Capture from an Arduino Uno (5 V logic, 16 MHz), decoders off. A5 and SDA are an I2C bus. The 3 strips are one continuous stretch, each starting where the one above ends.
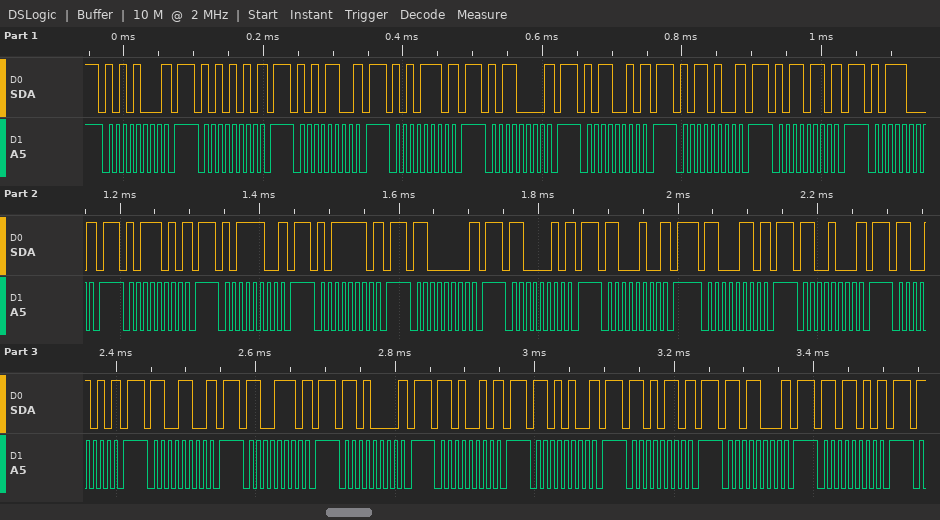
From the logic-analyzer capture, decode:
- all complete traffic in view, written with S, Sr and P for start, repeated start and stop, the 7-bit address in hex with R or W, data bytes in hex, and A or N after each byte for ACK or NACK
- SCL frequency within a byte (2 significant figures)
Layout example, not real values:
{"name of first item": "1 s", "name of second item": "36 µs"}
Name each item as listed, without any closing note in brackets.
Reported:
{"all complete traffic in view, written with S, Sr and P for start, repeated start and stop, the 7-bit address in hex with R or W, data bytes in hex, and A or N after each byte for ACK or NACK": "S 54W N P S 55W N P S 56W N P S 57W N P S 58W N P S 59W N P S 5AW N P S 5BW N P S 5CW N P S 5DW N P S 5EW N P S 5FW N P S 60W N P S 61W N P S 62W N P S 63W N P S 64W N P S 65W N P S 66W N P S 67W N P S 68W N P S 69W N P S 6AW N P S 6BW N P S 6CW N P S 6DW N P", "SCL frequency within a byte": "100 kHz"}
